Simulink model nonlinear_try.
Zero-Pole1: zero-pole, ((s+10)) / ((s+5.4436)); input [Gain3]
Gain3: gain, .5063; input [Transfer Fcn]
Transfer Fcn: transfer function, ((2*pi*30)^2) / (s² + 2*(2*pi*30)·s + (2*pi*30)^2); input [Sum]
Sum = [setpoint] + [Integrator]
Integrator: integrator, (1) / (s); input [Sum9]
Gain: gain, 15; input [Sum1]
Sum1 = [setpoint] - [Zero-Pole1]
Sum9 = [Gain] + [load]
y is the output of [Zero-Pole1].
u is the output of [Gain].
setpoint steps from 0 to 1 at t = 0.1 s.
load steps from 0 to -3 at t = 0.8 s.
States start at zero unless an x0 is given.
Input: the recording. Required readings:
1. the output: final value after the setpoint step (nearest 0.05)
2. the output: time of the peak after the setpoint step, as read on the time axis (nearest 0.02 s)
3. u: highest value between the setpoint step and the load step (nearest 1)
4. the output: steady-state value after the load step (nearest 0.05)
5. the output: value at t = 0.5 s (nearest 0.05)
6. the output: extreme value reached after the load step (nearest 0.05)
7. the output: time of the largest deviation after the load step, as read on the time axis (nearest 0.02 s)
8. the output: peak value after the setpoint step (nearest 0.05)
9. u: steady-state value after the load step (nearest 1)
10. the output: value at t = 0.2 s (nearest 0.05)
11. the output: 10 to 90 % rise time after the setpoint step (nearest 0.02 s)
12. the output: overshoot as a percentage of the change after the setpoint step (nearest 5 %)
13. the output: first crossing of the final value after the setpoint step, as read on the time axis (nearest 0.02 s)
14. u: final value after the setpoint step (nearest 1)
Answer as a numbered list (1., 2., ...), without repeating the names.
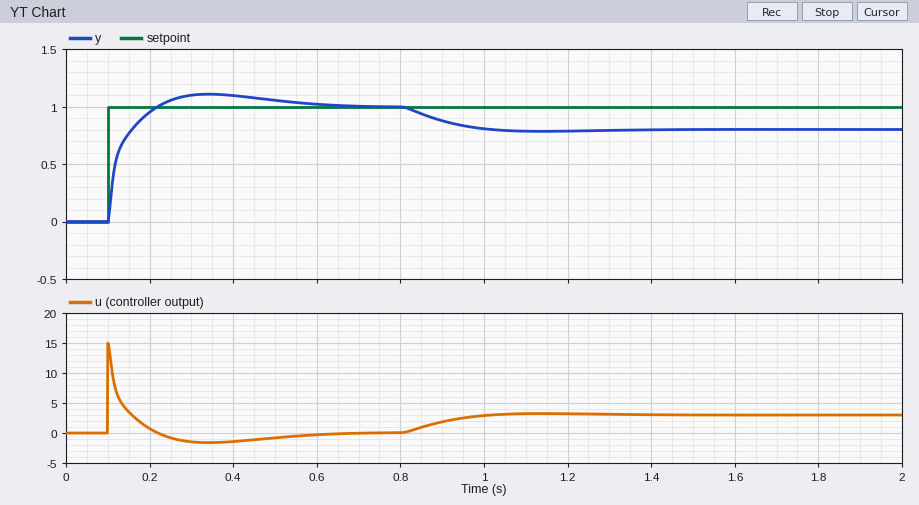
1. 1.00
2. 0.34 s
3. 15
4. 0.80
5. 1.05
6. 0.80
7. 1.14 s
8. 1.10
9. 3
10. 0.95
11. 0.08 s
12. 10 %
13. 0.22 s
14. 0
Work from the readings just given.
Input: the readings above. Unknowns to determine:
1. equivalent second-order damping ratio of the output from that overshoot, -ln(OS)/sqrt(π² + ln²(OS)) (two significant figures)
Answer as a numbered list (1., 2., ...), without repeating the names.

1. 0.59
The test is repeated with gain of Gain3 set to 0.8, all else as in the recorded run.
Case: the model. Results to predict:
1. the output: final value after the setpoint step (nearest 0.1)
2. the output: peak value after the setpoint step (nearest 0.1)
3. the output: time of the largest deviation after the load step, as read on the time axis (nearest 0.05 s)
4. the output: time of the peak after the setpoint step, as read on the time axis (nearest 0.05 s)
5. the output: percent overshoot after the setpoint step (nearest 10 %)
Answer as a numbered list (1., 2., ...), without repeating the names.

1. 1.0
2. 1.2
3. 1.05 s
4. 0.20 s
5. 20 %
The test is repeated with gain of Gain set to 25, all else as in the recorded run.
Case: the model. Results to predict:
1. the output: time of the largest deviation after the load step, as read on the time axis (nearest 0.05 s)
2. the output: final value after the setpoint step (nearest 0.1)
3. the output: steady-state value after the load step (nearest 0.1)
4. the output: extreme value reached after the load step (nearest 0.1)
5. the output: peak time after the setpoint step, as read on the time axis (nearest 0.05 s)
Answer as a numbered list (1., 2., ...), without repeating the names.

1. 1.05 s
2. 1.0
3. 0.9
4. 0.9
5. 0.25 s
